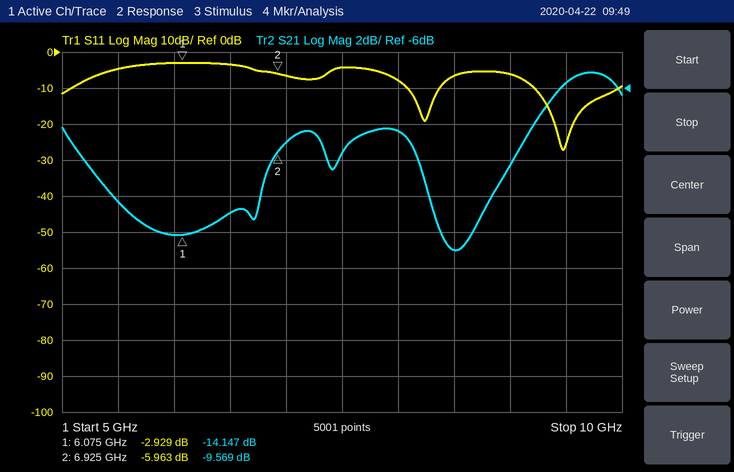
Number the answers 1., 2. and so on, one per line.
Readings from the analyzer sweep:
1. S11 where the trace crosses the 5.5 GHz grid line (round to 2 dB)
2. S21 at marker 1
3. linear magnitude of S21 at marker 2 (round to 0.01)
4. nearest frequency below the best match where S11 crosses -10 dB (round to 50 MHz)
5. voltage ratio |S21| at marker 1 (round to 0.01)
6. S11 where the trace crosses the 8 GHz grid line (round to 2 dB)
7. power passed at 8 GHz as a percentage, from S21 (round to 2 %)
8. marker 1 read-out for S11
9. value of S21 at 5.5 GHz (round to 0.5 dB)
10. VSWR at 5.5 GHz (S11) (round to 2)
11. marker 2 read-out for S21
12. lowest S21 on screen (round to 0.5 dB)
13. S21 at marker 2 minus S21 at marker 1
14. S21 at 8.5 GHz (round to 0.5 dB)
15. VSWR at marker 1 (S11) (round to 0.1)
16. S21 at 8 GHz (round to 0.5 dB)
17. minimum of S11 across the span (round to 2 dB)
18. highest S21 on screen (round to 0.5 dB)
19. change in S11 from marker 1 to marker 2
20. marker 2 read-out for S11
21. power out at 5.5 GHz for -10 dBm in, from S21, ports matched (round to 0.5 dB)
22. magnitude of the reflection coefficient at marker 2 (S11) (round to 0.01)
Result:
1. -4 dB
2. -14.147 dB
3. 0.33
4. 9.20 GHz
5. 0.20
6. -8 dB
7. 14 %
8. -2.929 dB
9. -12.5 dB
10. 4
11. -9.569 dB
12. -15.0 dB
13. 4.578 dB
14. -15.0 dB
15. 6.0
16. -8.5 dB
17. -28 dB
18. -5.0 dB
19. -3.034 dB
20. -5.963 dB
21. -22.5 dBm
22. 0.50
